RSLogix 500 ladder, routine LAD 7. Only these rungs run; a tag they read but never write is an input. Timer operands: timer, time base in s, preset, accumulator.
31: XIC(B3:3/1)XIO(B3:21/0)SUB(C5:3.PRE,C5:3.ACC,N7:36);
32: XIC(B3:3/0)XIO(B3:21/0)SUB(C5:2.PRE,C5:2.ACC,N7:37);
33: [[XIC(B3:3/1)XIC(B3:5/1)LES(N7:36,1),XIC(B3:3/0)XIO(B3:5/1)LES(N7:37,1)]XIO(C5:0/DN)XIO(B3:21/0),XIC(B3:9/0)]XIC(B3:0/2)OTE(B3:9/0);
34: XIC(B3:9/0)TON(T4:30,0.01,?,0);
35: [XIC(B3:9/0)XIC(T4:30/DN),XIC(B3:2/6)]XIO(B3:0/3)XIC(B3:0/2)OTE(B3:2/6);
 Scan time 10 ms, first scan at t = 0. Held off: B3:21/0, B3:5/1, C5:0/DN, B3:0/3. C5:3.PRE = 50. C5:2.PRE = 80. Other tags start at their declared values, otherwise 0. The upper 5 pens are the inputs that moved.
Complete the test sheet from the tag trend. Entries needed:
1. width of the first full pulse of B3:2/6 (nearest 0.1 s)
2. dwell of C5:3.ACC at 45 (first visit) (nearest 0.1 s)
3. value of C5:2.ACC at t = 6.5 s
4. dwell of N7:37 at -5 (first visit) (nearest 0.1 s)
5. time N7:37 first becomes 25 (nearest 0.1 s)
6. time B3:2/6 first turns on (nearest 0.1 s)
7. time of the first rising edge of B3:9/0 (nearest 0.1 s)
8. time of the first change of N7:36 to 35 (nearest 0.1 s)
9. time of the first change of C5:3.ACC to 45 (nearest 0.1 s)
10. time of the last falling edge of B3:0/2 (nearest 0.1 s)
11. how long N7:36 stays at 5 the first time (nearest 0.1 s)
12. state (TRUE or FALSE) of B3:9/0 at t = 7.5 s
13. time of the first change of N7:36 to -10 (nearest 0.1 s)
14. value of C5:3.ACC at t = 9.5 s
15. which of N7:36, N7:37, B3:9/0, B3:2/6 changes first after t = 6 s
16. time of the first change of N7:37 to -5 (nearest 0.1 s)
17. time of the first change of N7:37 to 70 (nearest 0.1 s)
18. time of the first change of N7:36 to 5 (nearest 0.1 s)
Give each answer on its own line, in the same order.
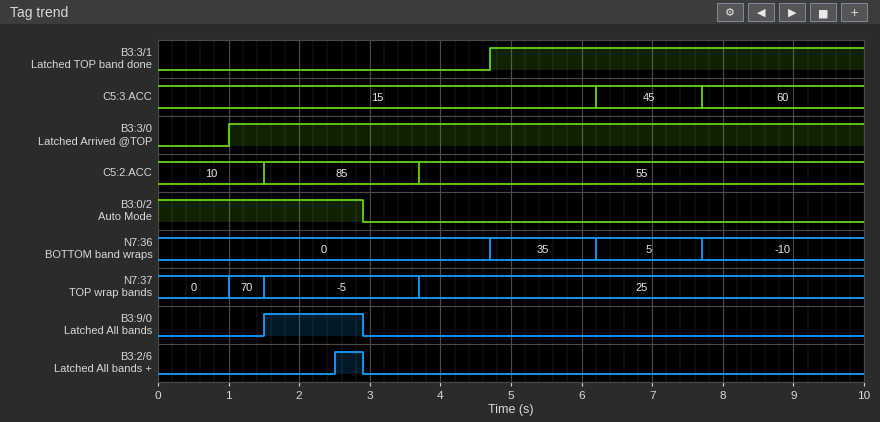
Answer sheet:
0.4 s
1.5 s
55
2.2 s
3.7 s
2.5 s
1.5 s
4.7 s
6.2 s
2.9 s
1.5 s
FALSE
7.7 s
60
N7:36
1.5 s
1.0 s
6.2 s
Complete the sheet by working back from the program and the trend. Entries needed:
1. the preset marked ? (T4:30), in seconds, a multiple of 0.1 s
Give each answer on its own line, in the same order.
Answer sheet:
1.0 s
